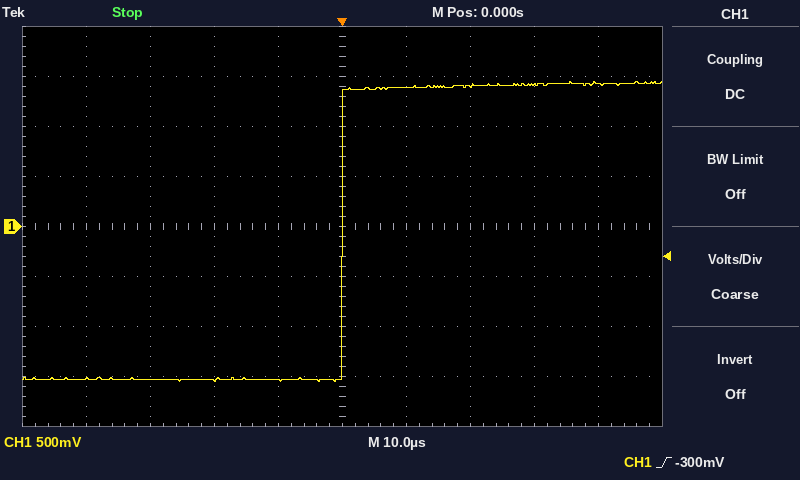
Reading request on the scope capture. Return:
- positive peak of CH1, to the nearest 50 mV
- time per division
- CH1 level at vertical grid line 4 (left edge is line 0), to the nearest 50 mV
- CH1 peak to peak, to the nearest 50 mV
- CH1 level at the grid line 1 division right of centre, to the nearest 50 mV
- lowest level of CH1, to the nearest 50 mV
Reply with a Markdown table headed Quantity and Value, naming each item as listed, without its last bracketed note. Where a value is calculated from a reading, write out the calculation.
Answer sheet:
| Quantity | Value |
|---|---|
| positive peak of CH1, to the nearest 50 mV | 1.45 V |
| time per division | 10 µs |
| CH1 level at vertical grid line 4 (left edge is line 0), to the nearest 50 mV | -1.55 V |
| CH1 peak to peak, to the nearest 50 mV | 1.45 V − (-1.55 V) = 3.00 V |
| CH1 level at the grid line 1 division right of centre, to the nearest 50 mV | 1.40 V |
| lowest level of CH1, to the nearest 50 mV | -1.55 V |
